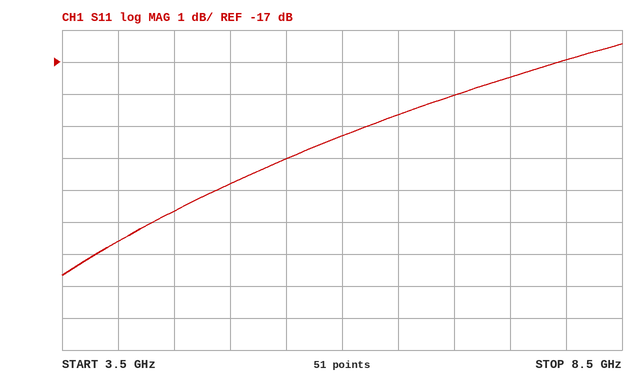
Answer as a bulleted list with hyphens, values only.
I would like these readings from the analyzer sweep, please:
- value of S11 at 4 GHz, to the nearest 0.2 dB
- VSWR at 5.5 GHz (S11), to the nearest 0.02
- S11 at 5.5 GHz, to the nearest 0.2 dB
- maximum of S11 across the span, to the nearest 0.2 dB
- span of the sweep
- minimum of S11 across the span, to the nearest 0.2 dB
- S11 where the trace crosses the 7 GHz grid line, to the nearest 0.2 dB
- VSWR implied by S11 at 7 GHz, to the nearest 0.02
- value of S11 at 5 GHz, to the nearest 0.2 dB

- -22.6 dB
- 1.22
- -20.0 dB
- -16.4 dB
- 5 GHz
- -23.6 dB
- -18.0 dB
- 1.28
- -20.8 dB
